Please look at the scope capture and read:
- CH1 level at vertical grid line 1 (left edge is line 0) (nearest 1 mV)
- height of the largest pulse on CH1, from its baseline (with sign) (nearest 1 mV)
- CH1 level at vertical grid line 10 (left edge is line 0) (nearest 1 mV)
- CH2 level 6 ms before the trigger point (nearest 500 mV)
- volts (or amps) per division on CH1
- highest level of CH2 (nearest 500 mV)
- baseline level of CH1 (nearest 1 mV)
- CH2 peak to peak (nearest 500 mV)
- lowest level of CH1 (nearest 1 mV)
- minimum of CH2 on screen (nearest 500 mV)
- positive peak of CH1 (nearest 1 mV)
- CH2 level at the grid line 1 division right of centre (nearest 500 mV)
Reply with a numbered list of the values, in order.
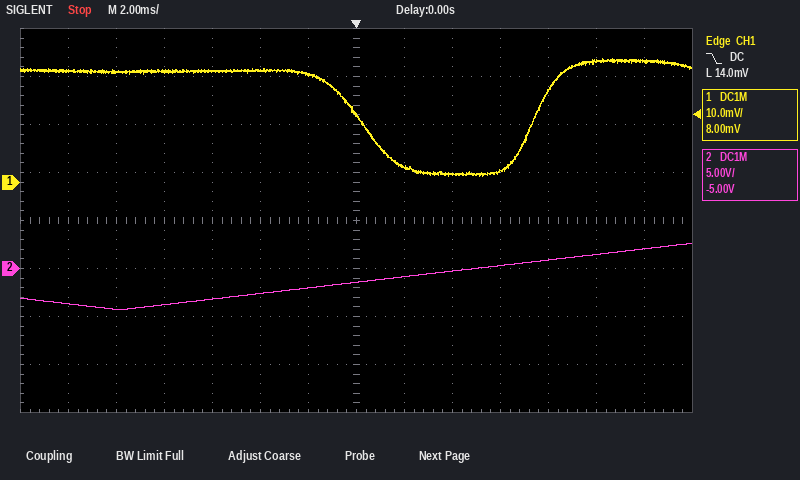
1. 23 mV
2. -22 mV
3. 2 mV
4. -3.0 V
5. 10 mV
6. 2.5 V
7. 23 mV
8. 7.0 V
9. 1 mV
10. -4.5 V
11. 26 mV
12. -1.0 V
